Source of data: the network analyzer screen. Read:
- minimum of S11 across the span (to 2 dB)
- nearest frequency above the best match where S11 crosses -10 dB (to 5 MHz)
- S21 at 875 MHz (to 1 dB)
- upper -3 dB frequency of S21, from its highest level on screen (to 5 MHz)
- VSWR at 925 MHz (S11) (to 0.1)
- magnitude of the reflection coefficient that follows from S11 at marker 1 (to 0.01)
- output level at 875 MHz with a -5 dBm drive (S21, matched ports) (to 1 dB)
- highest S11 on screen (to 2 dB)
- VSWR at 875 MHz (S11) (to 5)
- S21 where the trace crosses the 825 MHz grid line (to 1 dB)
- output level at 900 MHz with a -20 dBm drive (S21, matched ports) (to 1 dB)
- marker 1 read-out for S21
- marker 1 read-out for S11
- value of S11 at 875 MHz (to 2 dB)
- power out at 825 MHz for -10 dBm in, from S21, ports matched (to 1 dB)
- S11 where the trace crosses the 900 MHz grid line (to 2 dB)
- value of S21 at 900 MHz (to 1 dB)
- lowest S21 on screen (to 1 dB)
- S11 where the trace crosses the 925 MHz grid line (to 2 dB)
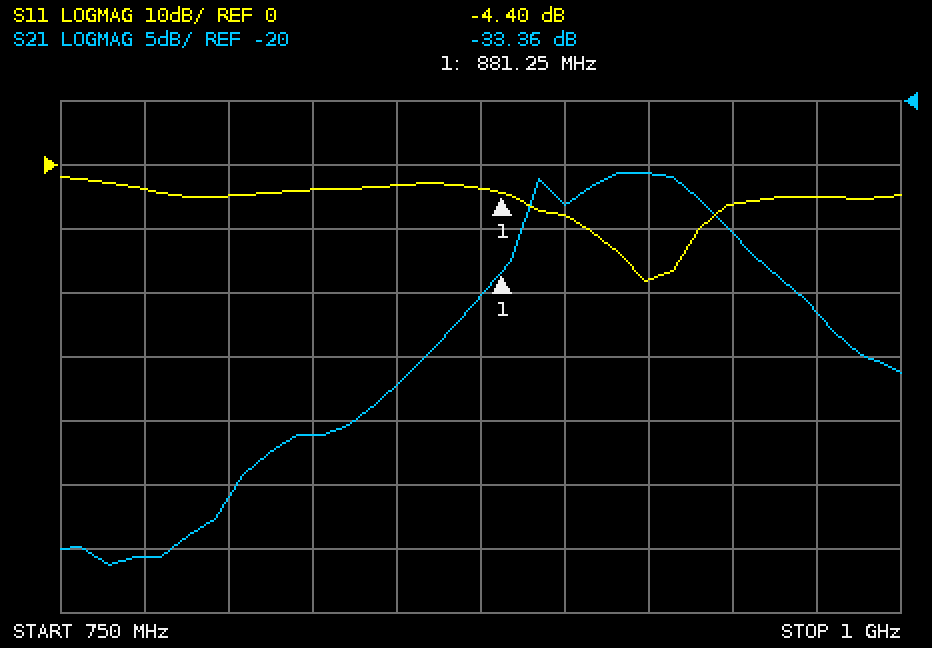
-18 dB
940 MHz
-35 dB
945 MHz
1.3
0.60
-40 dBm
-2 dB
5
-46 dB
-48 dBm
-33.36 dB
-4.40 dB
-4 dB
-56 dBm
-8 dB
-28 dB
-56 dB
-18 dB
